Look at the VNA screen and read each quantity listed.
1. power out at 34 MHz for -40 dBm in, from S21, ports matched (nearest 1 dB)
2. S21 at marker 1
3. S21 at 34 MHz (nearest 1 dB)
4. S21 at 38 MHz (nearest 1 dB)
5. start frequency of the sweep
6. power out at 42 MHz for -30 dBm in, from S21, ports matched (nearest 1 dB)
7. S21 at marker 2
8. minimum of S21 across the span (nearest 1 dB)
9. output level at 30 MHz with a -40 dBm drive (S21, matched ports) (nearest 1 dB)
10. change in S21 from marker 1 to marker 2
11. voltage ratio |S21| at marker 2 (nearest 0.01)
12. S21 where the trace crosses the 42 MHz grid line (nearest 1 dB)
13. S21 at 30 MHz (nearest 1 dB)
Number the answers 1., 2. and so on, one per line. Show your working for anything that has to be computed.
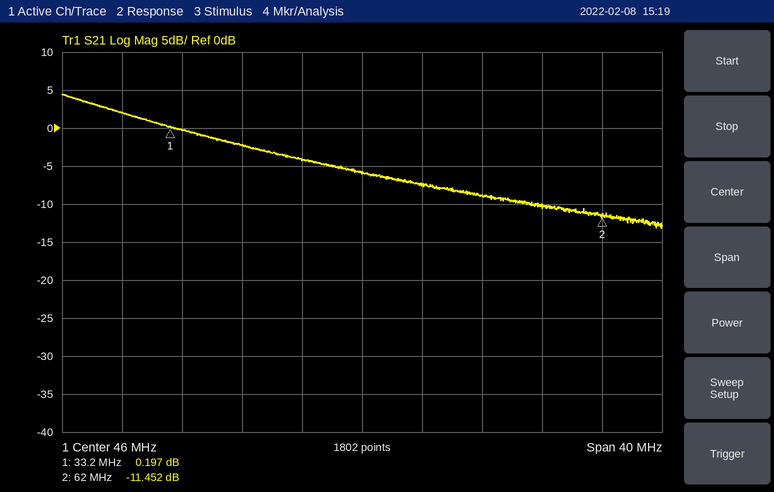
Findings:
1. -40 dBm + (0 dB) = -40 dBm
2. 0.197 dB
3. 0 dB
4. -2 dB
5. 26 MHz
6. -30 dBm + (-4 dB) = -34 dBm
7. -11.452 dB
8. -13 dB
9. -40 dBm + (2 dB) = -38 dBm
10. -11.452 − (0.197) = -11.649 dB
11. 10^(-11.452/20) ≈ 0.27
12. -4 dB
13. 2 dB
